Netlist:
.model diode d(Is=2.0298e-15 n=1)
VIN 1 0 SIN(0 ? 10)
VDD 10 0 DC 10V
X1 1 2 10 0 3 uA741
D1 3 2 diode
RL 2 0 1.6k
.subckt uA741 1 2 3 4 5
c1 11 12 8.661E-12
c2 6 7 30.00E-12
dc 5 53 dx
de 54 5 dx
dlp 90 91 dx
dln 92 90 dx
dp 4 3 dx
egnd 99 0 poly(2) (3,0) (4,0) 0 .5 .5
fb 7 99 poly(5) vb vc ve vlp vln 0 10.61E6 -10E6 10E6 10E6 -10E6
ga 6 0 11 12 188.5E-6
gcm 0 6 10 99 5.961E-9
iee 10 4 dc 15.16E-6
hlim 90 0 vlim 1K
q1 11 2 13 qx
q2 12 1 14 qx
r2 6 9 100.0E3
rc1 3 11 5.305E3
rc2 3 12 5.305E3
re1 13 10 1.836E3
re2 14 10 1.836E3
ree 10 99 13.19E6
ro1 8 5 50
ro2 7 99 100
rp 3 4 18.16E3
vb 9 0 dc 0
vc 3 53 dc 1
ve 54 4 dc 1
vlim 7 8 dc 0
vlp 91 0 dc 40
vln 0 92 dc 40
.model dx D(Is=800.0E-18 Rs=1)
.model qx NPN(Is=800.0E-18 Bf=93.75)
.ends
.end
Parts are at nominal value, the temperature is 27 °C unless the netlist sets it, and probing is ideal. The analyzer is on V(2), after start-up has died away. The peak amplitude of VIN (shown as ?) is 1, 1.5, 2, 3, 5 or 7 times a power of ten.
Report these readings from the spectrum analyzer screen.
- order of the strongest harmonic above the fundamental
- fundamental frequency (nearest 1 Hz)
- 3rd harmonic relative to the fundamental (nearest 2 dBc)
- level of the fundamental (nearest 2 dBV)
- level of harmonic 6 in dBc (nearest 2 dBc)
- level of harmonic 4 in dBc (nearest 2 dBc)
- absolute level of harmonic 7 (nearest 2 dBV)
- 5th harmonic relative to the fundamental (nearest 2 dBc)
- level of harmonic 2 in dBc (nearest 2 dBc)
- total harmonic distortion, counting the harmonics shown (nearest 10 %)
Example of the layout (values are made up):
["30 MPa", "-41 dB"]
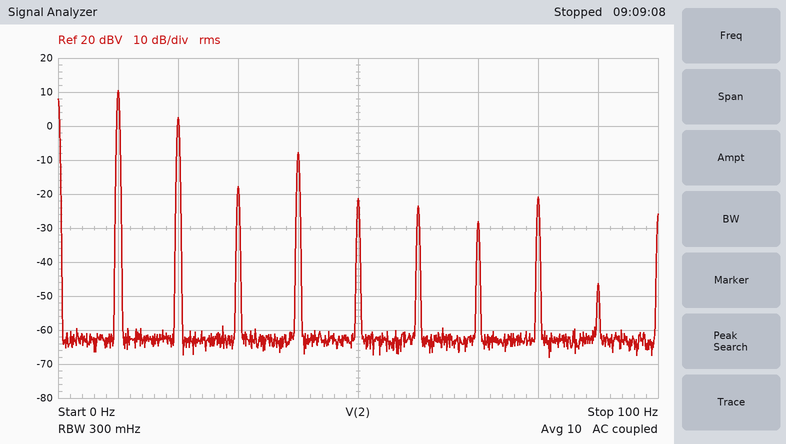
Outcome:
["2", "10 Hz", "-28 dBc", "10 dBV", "-34 dBc", "-18 dBc", "-28 dBV", "-32 dBc", "-8 dBc", "40 %"]
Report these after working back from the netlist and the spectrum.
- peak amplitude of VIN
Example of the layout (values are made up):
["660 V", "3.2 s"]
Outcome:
["10 V"]
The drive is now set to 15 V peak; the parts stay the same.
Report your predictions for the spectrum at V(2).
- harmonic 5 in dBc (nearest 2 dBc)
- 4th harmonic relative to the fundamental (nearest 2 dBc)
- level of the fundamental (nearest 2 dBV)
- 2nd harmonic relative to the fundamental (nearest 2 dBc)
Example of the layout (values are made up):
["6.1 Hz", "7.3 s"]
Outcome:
["-4 dBc", "-2 dBc", "0 dBV", "0 dBc"]
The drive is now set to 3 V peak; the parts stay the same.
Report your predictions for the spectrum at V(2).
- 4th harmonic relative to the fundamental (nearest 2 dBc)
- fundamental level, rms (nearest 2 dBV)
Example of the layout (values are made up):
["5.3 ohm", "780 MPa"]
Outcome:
["-22 dBc", "0 dBV"]
